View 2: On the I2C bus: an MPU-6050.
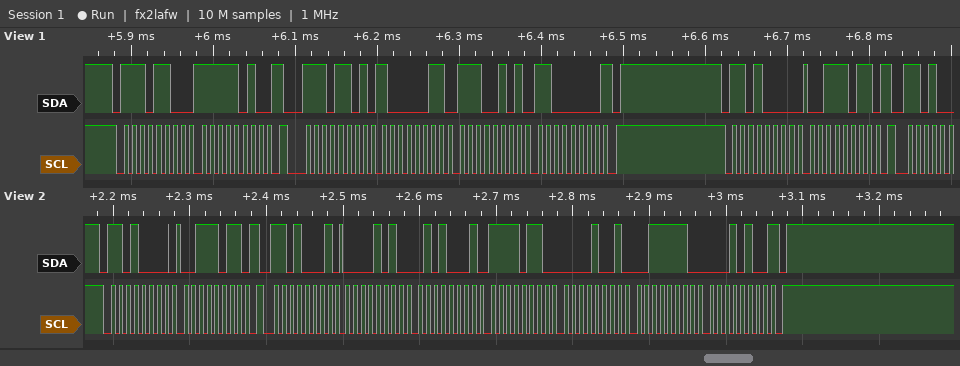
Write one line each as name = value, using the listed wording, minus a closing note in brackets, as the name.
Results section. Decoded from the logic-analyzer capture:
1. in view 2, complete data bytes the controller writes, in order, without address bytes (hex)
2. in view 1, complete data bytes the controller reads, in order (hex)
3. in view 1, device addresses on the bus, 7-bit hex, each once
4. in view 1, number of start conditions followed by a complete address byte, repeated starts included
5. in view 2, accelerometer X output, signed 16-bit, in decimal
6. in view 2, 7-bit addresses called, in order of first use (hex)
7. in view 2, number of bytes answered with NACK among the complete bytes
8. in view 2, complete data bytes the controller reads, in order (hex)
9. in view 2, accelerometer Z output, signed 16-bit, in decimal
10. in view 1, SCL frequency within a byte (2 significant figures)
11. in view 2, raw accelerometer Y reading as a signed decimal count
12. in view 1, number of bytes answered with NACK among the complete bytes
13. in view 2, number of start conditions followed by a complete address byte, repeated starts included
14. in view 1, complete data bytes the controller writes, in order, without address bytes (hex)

in view 2, complete data bytes the controller writes, in order, without address bytes = 3B
in view 1, complete data bytes the controller reads, in order = 83 E5 C0
in view 1, device addresses on the bus, 7-bit hex, each once = 0x76 0x68
in view 1, number of start conditions followed by a complete address byte, repeated starts included = 3
in view 2, accelerometer X output, signed 16-bit, in decimal = 2641
in view 2, 7-bit addresses called, in order of first use = 0x68
in view 2, number of bytes answered with NACK among the complete bytes = 1
in view 2, complete data bytes the controller reads, in order = 0A 51 F6 09 3E 14
in view 2, accelerometer Z output, signed 16-bit, in decimal = 15892
in view 1, SCL frequency within a byte = 100 kHz
in view 2, raw accelerometer Y reading as a signed decimal count = -2551
in view 1, number of bytes answered with NACK among the complete bytes = 1
in view 2, number of start conditions followed by a complete address byte, repeated starts included = 2
in view 1, complete data bytes the controller writes, in order, without address bytes = FA 3B
